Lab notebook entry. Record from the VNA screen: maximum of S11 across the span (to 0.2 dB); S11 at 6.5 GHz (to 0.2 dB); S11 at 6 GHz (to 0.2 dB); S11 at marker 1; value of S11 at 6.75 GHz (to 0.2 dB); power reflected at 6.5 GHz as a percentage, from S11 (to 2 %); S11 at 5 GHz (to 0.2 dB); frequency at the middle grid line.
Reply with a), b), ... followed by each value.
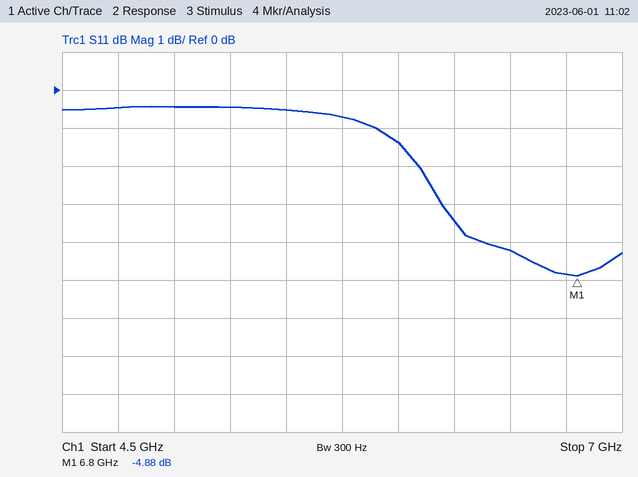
a) -0.4 dB
b) -4.2 dB
c) -1.4 dB
d) -4.88 dB
e) -4.8 dB
f) 38 %
g) -0.4 dB
h) 5.75 GHz
